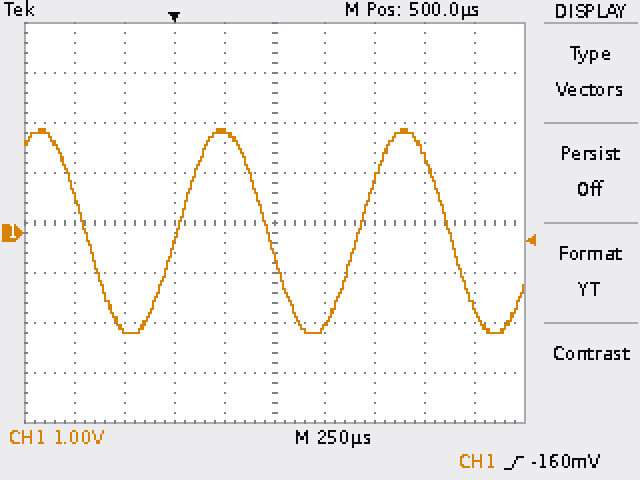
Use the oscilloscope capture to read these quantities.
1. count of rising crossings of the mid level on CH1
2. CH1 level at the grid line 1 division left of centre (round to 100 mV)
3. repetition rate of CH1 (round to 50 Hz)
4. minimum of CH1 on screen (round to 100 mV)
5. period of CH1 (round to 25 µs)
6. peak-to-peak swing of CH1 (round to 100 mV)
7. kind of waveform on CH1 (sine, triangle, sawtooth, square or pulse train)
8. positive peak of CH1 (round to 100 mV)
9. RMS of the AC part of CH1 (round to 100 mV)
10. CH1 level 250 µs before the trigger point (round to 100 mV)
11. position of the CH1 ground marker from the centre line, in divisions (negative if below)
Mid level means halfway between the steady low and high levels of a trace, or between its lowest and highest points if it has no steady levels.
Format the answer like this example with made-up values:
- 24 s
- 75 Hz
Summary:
- 2
- 2.0 V
- 1.10 kHz
- -2.0 V
- 900 µs
- 4.1 V
- sine
- 2.1 V
- 1.4 V
- -1.9 V
- -0.2 div
